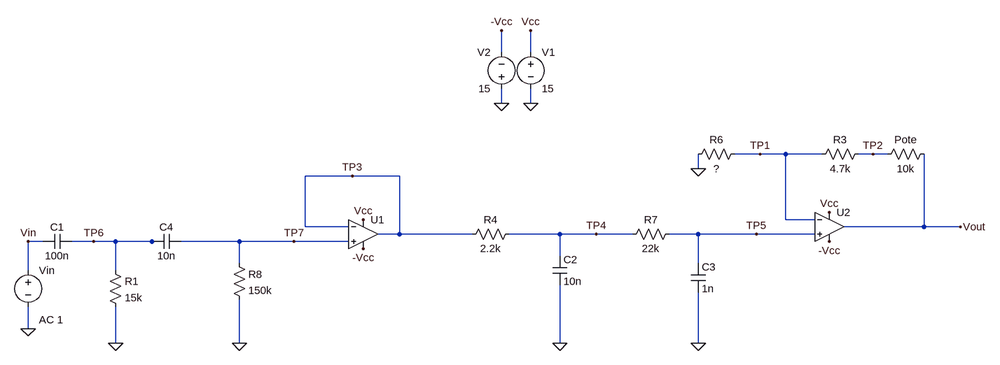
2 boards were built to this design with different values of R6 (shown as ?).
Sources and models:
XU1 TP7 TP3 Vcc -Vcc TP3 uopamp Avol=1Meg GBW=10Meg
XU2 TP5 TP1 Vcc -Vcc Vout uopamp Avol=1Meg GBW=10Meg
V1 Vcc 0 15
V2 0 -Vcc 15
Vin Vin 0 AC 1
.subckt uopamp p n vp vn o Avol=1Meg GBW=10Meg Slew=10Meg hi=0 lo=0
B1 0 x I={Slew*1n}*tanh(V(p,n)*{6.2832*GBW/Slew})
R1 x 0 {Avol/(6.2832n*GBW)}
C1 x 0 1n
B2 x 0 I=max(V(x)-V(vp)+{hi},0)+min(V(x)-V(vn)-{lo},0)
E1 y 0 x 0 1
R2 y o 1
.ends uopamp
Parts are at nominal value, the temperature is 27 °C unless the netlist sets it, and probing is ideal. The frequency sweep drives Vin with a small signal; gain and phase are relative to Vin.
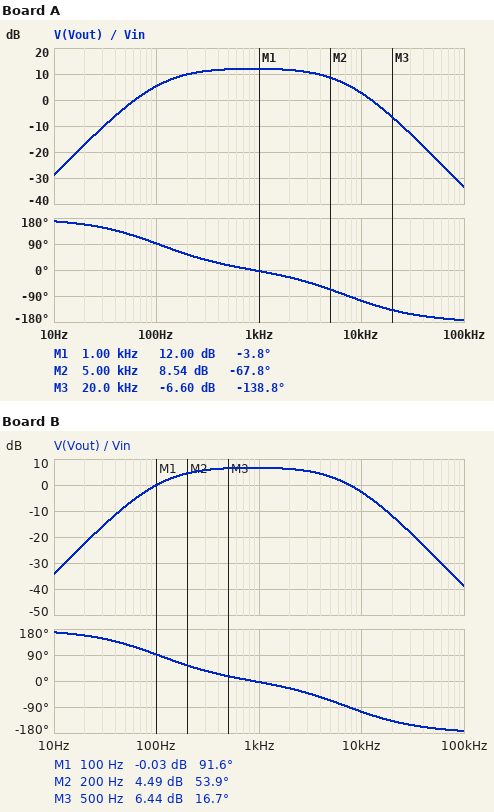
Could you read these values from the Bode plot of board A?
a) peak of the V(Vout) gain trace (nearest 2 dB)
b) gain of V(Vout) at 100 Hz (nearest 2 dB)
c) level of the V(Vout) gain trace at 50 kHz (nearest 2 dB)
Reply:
12 dB
6 dB
-22 dB
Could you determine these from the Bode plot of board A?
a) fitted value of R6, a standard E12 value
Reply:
4.7 kΩ
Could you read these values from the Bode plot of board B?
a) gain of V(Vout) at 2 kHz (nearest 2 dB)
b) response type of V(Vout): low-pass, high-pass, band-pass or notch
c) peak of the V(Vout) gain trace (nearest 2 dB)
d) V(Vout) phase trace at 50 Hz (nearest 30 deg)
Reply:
6 dB
band-pass
6 dB
120 deg
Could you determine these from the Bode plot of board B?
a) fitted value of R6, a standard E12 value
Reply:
12 kΩ
